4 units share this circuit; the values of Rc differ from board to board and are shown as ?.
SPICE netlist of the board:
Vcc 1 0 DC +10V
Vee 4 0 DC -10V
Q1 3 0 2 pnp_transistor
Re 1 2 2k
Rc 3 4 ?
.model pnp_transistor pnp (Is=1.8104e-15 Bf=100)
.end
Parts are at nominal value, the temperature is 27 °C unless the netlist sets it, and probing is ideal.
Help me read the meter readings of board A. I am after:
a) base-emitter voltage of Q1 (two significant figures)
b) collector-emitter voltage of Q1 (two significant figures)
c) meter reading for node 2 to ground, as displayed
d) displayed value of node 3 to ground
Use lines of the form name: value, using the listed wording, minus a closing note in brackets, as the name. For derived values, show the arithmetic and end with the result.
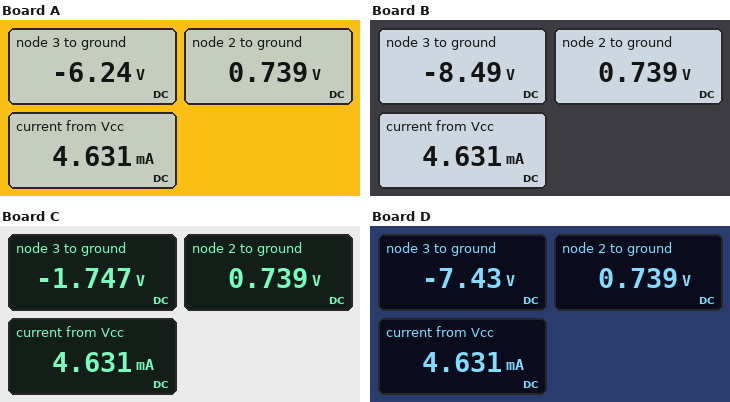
base-emitter voltage of Q1: 0 V - 739 mV = -740 mV
collector-emitter voltage of Q1: -6.24 V - 739 mV = -7.0 V
meter reading for node 2 to ground, as displayed: 0.739 V
displayed value of node 3 to ground: -6.24 V
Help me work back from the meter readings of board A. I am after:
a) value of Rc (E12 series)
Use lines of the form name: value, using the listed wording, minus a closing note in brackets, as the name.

value of Rc: 820 Ω
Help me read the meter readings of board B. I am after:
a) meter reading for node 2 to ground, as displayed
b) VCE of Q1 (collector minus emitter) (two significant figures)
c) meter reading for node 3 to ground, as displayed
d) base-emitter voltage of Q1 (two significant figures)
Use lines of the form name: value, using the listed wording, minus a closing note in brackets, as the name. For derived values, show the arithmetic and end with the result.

meter reading for node 2 to ground, as displayed: 0.739 V
VCE of Q1 (collector minus emitter): -8.49 V - 739 mV = -9.2 V
meter reading for node 3 to ground, as displayed: -8.49 V
base-emitter voltage of Q1: 0 V - 739 mV = -740 mV
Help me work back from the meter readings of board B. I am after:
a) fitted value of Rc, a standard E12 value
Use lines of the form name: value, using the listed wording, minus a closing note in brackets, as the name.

fitted value of Rc, a standard E12 value: 330 Ω
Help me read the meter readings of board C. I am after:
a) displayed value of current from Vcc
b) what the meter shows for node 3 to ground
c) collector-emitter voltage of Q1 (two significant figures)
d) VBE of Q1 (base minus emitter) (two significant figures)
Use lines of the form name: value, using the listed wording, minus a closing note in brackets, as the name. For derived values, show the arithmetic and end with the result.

displayed value of current from Vcc: 4.631 mA
what the meter shows for node 3 to ground: -1.747 V
collector-emitter voltage of Q1: -1.747 V - 739 mV = -2.5 V
VBE of Q1 (base minus emitter): 0 V - 739 mV = -740 mV
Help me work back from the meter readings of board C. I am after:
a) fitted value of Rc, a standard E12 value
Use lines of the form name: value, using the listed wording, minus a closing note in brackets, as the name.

fitted value of Rc, a standard E12 value: 1.8 kΩ
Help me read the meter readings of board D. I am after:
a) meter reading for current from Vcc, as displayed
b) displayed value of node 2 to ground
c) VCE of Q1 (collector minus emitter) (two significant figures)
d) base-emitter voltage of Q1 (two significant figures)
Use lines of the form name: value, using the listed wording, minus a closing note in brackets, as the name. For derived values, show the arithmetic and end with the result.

meter reading for current from Vcc, as displayed: 4.631 mA
displayed value of node 2 to ground: 0.739 V
VCE of Q1 (collector minus emitter): -7.43 V - 739 mV = -8.2 V
base-emitter voltage of Q1: 0 V - 739 mV = -740 mV
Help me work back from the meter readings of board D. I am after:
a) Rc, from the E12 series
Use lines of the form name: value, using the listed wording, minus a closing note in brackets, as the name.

Rc, from the E12 series: 560 Ω
